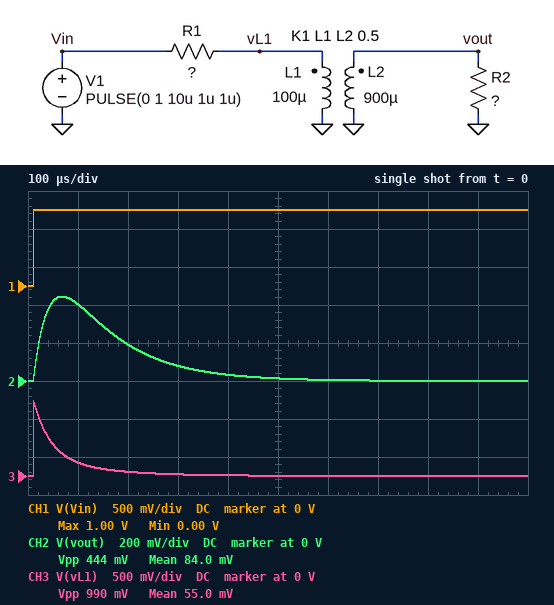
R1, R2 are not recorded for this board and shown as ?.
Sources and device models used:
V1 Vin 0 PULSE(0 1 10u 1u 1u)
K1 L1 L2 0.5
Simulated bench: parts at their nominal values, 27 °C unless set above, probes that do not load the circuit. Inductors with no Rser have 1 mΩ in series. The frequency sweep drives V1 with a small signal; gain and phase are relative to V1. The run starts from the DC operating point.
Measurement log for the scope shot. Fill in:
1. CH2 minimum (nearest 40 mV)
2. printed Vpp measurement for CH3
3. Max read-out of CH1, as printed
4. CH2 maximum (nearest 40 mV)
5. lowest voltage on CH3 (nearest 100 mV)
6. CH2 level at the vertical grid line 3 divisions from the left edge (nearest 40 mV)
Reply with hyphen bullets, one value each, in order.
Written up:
- 0 V
- 990 mV
- 1.00 V
- 440 mV
- 0 V
- 80 mV
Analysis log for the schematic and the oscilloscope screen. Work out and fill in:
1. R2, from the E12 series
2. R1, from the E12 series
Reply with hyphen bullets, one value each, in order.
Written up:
- 10 Ω
- 1.8 Ω
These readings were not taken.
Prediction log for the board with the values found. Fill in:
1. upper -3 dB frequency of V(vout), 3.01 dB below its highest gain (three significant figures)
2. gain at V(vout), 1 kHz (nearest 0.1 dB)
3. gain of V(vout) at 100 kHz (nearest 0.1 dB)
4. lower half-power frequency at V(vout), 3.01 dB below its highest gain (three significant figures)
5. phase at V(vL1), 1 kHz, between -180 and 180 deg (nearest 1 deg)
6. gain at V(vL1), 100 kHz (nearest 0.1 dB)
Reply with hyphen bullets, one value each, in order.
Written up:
- 7.13 kHz
- -7.6 dB
- -29.0 dB
- 948 Hz
- 66 deg
- 0 dB
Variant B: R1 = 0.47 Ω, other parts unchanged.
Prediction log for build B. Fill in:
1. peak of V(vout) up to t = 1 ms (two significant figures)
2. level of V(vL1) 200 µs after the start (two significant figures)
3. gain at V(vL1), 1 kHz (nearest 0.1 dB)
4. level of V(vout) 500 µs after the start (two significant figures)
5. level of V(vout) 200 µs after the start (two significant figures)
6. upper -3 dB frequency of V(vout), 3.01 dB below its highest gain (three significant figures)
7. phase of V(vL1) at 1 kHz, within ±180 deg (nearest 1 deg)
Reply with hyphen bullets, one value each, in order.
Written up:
- 830 mV
- 390 mV
- -2.6 dB
- 230 mV
- 720 mV
- 3.82 kHz
- 36 deg
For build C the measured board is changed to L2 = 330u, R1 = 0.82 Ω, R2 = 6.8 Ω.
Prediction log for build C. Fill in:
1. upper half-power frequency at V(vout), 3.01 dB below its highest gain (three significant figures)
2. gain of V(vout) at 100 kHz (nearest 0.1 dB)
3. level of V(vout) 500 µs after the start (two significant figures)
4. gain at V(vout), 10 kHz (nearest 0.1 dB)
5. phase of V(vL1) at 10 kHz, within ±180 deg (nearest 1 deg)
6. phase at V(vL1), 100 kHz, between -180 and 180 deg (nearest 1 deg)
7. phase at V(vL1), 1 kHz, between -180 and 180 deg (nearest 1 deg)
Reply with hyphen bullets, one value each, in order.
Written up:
- 6.94 kHz
- -28.0 dB
- 30 mV
- -9.0 dB
- 9 deg
- 1 deg
- 50 deg
